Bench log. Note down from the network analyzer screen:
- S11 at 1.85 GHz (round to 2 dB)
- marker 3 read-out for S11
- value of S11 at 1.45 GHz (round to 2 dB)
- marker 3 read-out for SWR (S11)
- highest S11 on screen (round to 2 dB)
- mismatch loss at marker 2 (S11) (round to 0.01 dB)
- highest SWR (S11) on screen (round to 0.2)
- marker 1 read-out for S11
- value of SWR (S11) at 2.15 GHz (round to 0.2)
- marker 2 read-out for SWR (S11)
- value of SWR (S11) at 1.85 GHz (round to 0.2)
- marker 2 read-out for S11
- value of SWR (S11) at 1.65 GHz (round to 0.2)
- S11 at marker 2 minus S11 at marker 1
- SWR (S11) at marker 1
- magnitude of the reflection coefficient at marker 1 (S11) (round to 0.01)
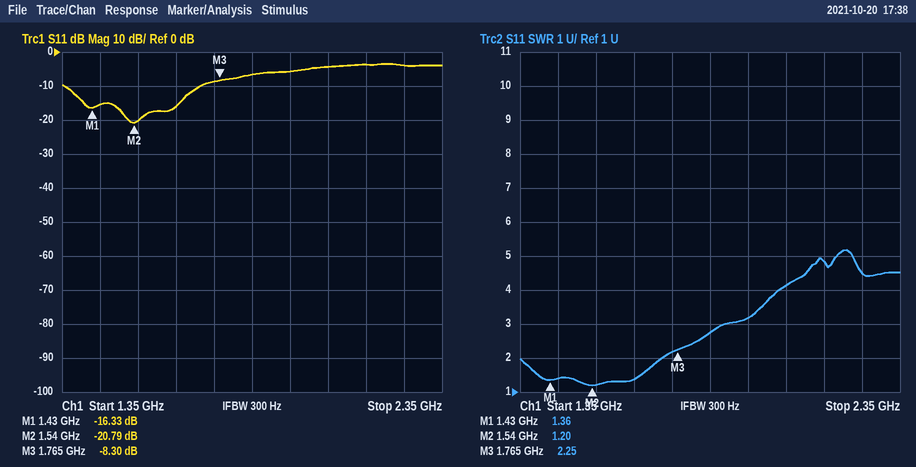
-6 dB
-8.30 dB
-16 dB
2.25
-4 dB
0.04 dB
5.2
-16.33 dB
4.8
1.20
2.8
-20.79 dB
1.4
-4.46 dB
1.36
0.15
